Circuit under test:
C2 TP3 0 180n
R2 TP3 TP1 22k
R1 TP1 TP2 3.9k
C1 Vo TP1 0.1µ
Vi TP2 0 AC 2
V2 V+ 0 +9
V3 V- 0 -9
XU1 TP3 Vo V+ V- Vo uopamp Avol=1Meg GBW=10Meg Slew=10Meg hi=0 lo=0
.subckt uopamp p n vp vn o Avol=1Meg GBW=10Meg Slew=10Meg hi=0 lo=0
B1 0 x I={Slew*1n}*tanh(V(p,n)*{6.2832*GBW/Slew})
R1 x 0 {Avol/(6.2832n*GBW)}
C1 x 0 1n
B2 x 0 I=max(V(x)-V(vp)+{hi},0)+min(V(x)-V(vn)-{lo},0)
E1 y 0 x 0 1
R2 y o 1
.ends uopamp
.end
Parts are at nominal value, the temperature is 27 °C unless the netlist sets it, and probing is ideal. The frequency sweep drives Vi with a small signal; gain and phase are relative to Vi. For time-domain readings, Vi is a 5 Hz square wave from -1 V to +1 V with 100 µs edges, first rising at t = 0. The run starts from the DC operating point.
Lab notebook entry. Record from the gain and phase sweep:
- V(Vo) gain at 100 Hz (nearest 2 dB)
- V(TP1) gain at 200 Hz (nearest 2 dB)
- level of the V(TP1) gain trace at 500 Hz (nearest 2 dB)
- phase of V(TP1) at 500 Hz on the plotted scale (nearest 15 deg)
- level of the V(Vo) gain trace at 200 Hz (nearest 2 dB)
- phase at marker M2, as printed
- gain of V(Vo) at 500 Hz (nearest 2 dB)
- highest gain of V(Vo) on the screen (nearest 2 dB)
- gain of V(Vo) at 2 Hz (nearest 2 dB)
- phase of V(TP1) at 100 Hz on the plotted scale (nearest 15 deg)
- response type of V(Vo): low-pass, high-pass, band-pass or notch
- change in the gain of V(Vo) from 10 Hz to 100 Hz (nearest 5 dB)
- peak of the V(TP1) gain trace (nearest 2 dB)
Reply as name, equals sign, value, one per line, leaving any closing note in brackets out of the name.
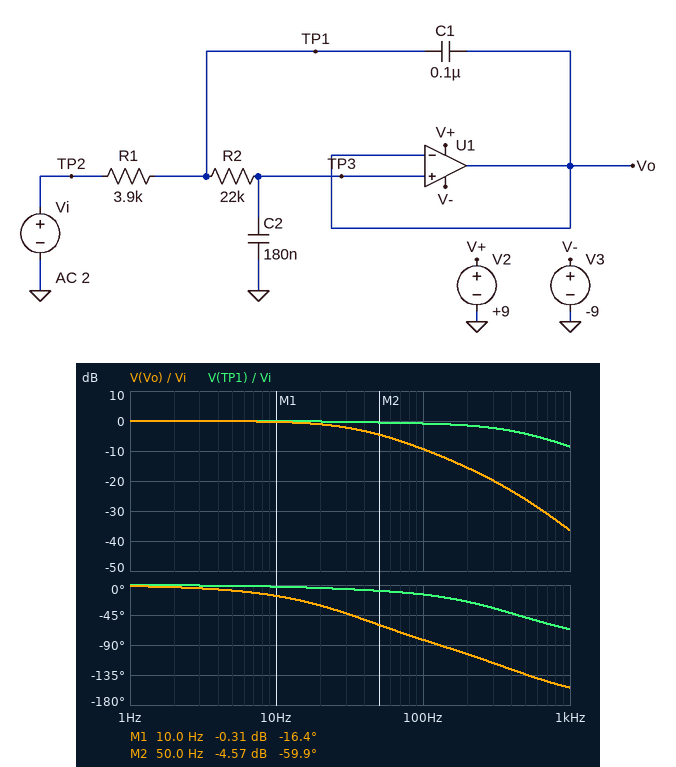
V(Vo) gain at 100 Hz = -10 dB
V(TP1) gain at 200 Hz = -2 dB
level of the V(TP1) gain trace at 500 Hz = -4 dB
phase of V(TP1) at 500 Hz on the plotted scale = -45 deg
level of the V(Vo) gain trace at 200 Hz = -16 dB
phase at marker M2, as printed = -59.9 deg
gain of V(Vo) at 500 Hz = -26 dB
highest gain of V(Vo) on the screen = 0 dB
gain of V(Vo) at 2 Hz = 0 dB
phase of V(TP1) at 100 Hz on the plotted scale = -15 deg
response type of V(Vo): low-pass, high-pass, band-pass or notch = low-pass
change in the gain of V(Vo) from 10 Hz to 100 Hz = -10 dB
peak of the V(TP1) gain trace = 0 dB
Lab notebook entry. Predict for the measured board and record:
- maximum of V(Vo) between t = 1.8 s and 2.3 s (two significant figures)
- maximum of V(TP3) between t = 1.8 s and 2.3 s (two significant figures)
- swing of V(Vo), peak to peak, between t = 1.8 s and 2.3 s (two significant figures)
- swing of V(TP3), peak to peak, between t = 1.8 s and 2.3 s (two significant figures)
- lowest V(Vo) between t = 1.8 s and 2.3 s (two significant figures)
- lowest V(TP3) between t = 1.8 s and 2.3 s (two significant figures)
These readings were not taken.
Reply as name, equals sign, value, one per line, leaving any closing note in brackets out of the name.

maximum of V(Vo) between t = 1.8 s and 2.3 s = 1.0 V
maximum of V(TP3) between t = 1.8 s and 2.3 s = 1.0 V
swing of V(Vo), peak to peak, between t = 1.8 s and 2.3 s = 2.0 V
swing of V(TP3), peak to peak, between t = 1.8 s and 2.3 s = 2.0 V
lowest V(Vo) between t = 1.8 s and 2.3 s = -1.0 V
lowest V(TP3) between t = 1.8 s and 2.3 s = -1.0 V
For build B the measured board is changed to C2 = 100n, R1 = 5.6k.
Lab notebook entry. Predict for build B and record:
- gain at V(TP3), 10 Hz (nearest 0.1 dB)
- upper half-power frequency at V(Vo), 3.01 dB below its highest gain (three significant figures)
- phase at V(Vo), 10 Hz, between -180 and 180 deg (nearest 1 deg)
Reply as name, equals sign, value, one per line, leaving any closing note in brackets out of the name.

gain at V(TP3), 10 Hz = -0.1 dB
upper half-power frequency at V(Vo), 3.01 dB below its highest gain = 68.3 Hz
phase at V(Vo), 10 Hz, between -180 and 180 deg = -10 deg
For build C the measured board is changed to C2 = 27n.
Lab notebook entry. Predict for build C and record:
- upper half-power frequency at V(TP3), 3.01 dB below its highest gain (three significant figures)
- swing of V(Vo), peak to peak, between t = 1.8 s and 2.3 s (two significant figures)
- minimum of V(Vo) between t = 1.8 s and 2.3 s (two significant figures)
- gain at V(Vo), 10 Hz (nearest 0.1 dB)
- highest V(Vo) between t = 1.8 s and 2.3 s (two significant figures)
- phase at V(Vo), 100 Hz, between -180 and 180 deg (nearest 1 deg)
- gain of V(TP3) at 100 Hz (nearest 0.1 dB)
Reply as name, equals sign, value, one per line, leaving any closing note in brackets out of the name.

upper half-power frequency at V(TP3), 3.01 dB below its highest gain = 322 Hz
swing of V(Vo), peak to peak, between t = 1.8 s and 2.3 s = 2.2 V
minimum of V(Vo) between t = 1.8 s and 2.3 s = -1.1 V
gain at V(Vo), 10 Hz = 0 dB
highest V(Vo) between t = 1.8 s and 2.3 s = 1.1 V
phase at V(Vo), 100 Hz, between -180 and 180 deg = -26 deg
gain of V(TP3) at 100 Hz = -0.1 dB
